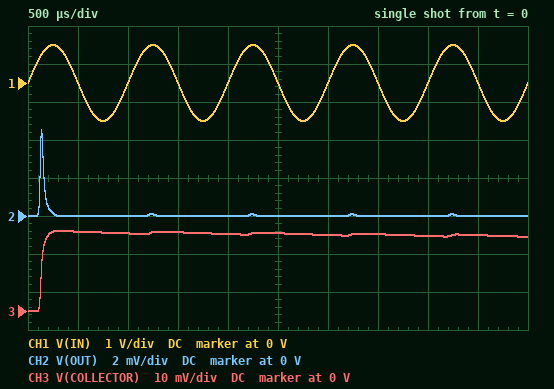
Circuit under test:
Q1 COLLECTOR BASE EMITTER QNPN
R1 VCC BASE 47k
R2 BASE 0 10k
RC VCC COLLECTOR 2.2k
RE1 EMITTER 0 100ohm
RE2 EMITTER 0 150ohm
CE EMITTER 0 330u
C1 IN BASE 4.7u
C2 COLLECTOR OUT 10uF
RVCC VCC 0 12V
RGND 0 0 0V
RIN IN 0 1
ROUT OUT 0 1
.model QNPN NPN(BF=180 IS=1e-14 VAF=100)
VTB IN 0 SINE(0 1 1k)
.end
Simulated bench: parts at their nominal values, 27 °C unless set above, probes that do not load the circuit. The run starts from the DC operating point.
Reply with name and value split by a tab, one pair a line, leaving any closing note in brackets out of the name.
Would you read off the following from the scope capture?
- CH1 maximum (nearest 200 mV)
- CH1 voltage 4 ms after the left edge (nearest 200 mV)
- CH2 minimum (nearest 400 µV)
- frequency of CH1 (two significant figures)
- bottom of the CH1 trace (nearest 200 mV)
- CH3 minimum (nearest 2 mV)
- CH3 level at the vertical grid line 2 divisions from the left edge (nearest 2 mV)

CH1 maximum	1.0 V
CH1 voltage 4 ms after the left edge	0 V
CH2 minimum	0 V
frequency of CH1	1.0 kHz
bottom of the CH1 trace	-1.0 V
CH3 minimum	0 V
CH3 level at the vertical grid line 2 divisions from the left edge	20 mV
